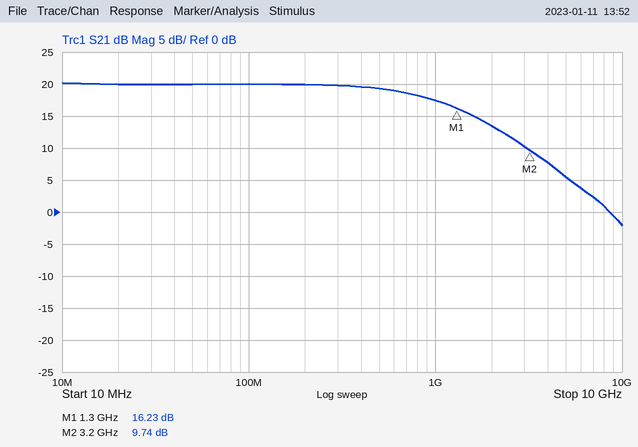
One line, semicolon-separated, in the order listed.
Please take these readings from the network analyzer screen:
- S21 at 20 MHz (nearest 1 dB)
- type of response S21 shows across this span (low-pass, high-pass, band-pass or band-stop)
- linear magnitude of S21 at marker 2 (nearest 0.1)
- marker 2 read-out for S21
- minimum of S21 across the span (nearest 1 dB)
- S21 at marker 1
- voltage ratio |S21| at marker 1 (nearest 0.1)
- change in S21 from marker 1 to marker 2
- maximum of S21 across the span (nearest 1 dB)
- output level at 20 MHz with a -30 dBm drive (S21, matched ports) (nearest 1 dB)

20 dB; low-pass; 3.1; 9.74 dB; -2 dB; 16.23 dB; 6.5; -6.49 dB; 20 dB; -10 dBm
